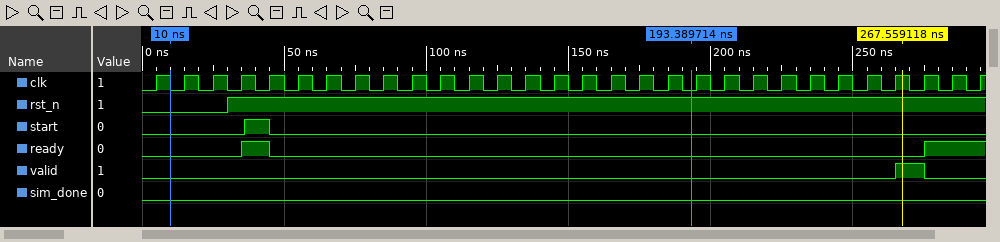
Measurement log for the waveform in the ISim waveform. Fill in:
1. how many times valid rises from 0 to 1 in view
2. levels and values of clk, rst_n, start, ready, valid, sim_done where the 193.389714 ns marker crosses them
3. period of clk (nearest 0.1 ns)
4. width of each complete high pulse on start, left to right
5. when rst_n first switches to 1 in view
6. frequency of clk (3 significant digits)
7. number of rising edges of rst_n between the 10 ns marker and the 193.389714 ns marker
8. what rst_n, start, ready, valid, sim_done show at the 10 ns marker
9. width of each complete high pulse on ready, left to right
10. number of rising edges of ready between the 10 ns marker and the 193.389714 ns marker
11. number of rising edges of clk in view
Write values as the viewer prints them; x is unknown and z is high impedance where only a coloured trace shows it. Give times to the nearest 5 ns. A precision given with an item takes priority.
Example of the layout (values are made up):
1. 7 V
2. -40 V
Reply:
1. 1
2. clk=0, rst_n=1, start=0, ready=0, valid=0, sim_done=0
3. 10 ns
4. 10 ns
5. 30 ns
6. 100 MHz
7. 1
8. rst_n=0, start=0, ready=0, valid=0, sim_done=0
9. 10 ns
10. 1
11. 30
